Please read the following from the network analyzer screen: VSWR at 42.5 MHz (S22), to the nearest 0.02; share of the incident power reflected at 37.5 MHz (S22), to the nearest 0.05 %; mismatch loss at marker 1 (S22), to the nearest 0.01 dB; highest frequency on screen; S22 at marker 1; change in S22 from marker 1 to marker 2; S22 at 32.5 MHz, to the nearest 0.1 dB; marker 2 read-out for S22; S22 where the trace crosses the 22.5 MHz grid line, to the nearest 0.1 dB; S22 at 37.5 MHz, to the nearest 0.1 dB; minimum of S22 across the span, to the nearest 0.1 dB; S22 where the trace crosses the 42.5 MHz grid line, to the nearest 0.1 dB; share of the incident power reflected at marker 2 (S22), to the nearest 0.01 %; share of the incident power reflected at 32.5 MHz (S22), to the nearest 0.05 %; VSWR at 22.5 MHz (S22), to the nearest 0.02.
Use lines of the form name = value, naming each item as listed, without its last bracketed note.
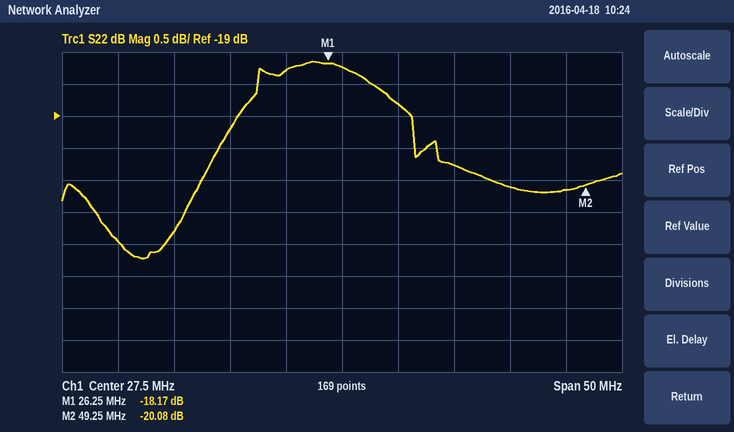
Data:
VSWR at 42.5 MHz (S22), to the nearest 0.02 = 1.22
share of the incident power reflected at 37.5 MHz (S22), to the nearest 0.05 % = 1.05 %
mismatch loss at marker 1 (S22), to the nearest 0.01 dB = 0.07 dB
highest frequency on screen = 52.5 MHz
S22 at marker 1 = -18.17 dB
change in S22 from marker 1 to marker 2 = -1.91 dB
S22 at 32.5 MHz, to the nearest 0.1 dB = -18.8 dB
marker 2 read-out for S22 = -20.08 dB
S22 where the trace crosses the 22.5 MHz grid line, to the nearest 0.1 dB = -18.3 dB
S22 at 37.5 MHz, to the nearest 0.1 dB = -19.8 dB
minimum of S22 across the span, to the nearest 0.1 dB = -21.2 dB
S22 where the trace crosses the 42.5 MHz grid line, to the nearest 0.1 dB = -20.1 dB
share of the incident power reflected at marker 2 (S22), to the nearest 0.01 % = 0.98 %
share of the incident power reflected at 32.5 MHz (S22), to the nearest 0.05 % = 1.30 %
VSWR at 22.5 MHz (S22), to the nearest 0.02 = 1.28
